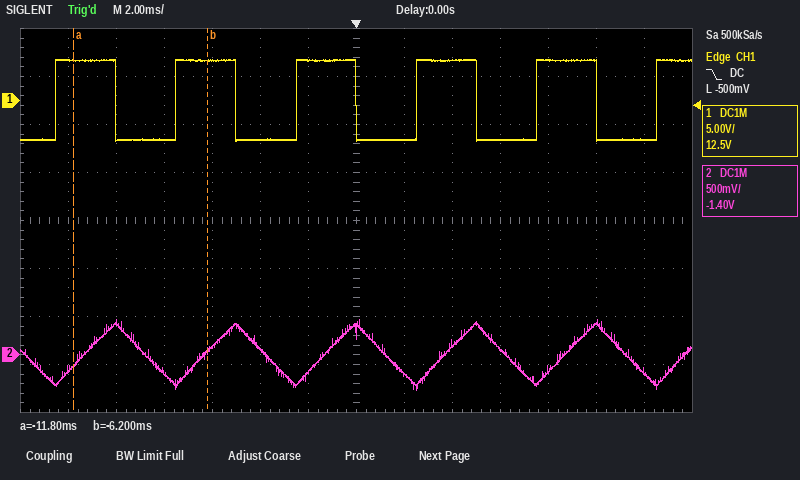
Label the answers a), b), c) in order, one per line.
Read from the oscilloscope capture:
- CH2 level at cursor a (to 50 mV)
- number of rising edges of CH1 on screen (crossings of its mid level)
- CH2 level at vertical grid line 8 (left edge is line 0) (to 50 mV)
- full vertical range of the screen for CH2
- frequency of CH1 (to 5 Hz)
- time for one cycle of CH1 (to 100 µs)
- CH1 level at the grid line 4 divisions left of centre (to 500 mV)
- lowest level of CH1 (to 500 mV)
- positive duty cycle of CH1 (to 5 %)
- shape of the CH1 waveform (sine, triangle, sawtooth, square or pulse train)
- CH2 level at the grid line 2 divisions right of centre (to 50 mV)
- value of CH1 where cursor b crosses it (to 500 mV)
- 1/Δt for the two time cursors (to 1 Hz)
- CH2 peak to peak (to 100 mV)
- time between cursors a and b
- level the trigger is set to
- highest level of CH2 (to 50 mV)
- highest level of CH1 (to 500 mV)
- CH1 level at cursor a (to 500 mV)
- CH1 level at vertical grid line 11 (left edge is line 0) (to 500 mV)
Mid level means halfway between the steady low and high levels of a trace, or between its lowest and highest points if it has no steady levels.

a) -100 mV
b) 6
c) -200 mV
d) 4 V
e) 200 Hz
f) 5.0 ms
g) -4.0 V
h) -4.5 V
i) 50 %
j) square
k) 100 mV
l) 4.0 V
m) 179 Hz
n) 700 mV
o) 5.6 ms
p) -500 mV
q) 350 mV
r) 4.5 V
s) 4.0 V
t) 4.0 V
